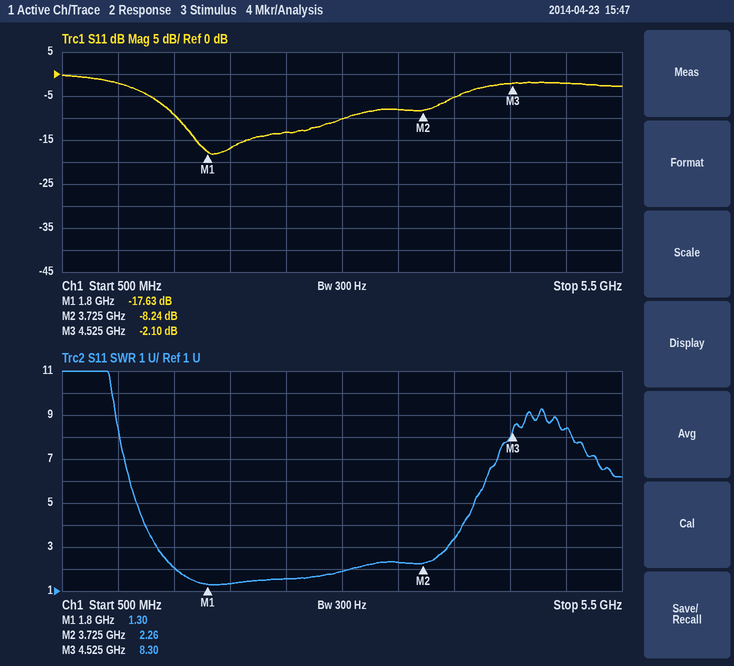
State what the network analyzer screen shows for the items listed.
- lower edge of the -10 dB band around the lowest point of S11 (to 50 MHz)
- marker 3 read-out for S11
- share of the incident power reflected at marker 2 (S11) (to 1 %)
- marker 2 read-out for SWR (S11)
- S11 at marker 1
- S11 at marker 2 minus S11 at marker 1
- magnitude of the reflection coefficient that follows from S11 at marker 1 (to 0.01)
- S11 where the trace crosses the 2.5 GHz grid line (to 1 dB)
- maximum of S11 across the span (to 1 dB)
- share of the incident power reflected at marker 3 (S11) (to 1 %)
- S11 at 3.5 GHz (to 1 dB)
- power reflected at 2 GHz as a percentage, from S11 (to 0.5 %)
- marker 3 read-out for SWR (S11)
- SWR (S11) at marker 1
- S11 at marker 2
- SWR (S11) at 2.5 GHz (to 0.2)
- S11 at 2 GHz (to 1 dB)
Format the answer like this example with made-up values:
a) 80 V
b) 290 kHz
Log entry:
a) 1.55 GHz
b) -2.10 dB
c) 15 %
d) 2.26
e) -17.63 dB
f) 9.39 dB
g) 0.13
h) -13 dB
i) 0 dB
j) 62 %
k) -8 dB
l) 2.0 %
m) 8.30
n) 1.30
o) -8.24 dB
p) 1.6
q) -17 dB
